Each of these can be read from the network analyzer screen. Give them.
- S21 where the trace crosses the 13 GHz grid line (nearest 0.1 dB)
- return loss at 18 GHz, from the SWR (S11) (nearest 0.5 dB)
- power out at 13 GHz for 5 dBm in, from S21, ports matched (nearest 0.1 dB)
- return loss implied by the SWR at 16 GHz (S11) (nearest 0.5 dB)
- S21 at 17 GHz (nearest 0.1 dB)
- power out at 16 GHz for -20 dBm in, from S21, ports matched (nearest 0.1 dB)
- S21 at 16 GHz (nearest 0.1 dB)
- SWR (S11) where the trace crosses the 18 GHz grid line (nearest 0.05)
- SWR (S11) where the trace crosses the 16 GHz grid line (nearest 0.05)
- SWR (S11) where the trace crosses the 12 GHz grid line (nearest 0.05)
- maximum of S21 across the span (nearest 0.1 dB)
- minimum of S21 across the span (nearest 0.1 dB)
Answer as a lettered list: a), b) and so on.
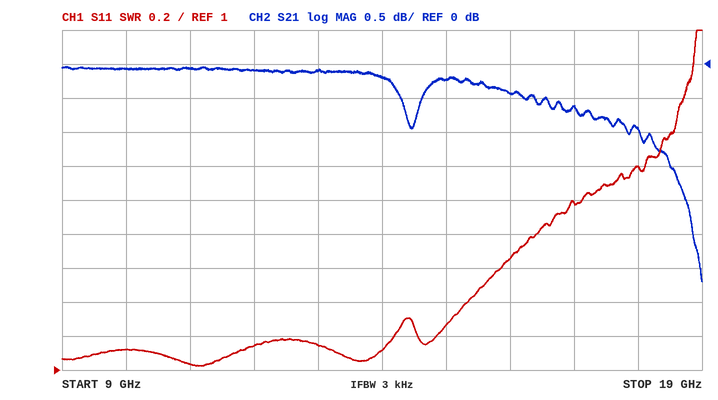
a) -0.1 dB
b) 8.5 dB
c) 4.9 dBm
d) 12.0 dB
e) -0.6 dB
f) -20.4 dBm
g) -0.4 dB
h) 2.20
i) 1.65
j) 1.15
k) 0.0 dB
l) -3.2 dB
